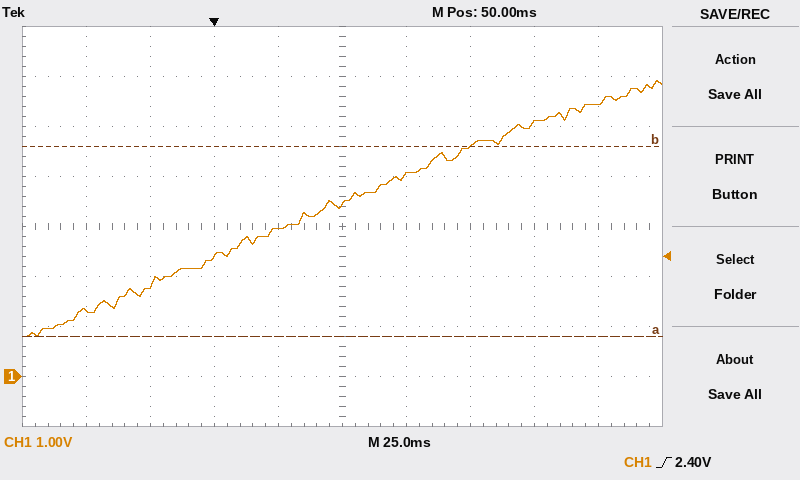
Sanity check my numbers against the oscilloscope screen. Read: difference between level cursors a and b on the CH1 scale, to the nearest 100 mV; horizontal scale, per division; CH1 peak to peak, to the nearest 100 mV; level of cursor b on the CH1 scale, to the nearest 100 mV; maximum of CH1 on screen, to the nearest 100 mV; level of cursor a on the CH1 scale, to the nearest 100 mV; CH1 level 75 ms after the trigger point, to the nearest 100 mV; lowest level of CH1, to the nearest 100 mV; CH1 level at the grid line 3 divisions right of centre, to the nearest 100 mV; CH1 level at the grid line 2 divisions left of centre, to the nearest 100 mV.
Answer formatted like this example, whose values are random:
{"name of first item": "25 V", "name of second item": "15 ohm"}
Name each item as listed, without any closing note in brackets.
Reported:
{"difference between level cursors a and b on the CH1 scale, to the nearest 100 mV": "3.8 V", "horizontal scale, per division": "25 ms", "CH1 peak to peak, to the nearest 100 mV": "5.1 V", "level of cursor b on the CH1 scale, to the nearest 100 mV": "4.6 V", "maximum of CH1 on screen, to the nearest 100 mV": "5.9 V", "level of cursor a on the CH1 scale, to the nearest 100 mV": "800 mV", "CH1 level 75 ms after the trigger point, to the nearest 100 mV": "4.0 V", "lowest level of CH1, to the nearest 100 mV": "800 mV", "CH1 level at the grid line 3 divisions right of centre, to the nearest 100 mV": "5.1 V", "CH1 level at the grid line 2 divisions left of centre, to the nearest 100 mV": "2.4 V"}
